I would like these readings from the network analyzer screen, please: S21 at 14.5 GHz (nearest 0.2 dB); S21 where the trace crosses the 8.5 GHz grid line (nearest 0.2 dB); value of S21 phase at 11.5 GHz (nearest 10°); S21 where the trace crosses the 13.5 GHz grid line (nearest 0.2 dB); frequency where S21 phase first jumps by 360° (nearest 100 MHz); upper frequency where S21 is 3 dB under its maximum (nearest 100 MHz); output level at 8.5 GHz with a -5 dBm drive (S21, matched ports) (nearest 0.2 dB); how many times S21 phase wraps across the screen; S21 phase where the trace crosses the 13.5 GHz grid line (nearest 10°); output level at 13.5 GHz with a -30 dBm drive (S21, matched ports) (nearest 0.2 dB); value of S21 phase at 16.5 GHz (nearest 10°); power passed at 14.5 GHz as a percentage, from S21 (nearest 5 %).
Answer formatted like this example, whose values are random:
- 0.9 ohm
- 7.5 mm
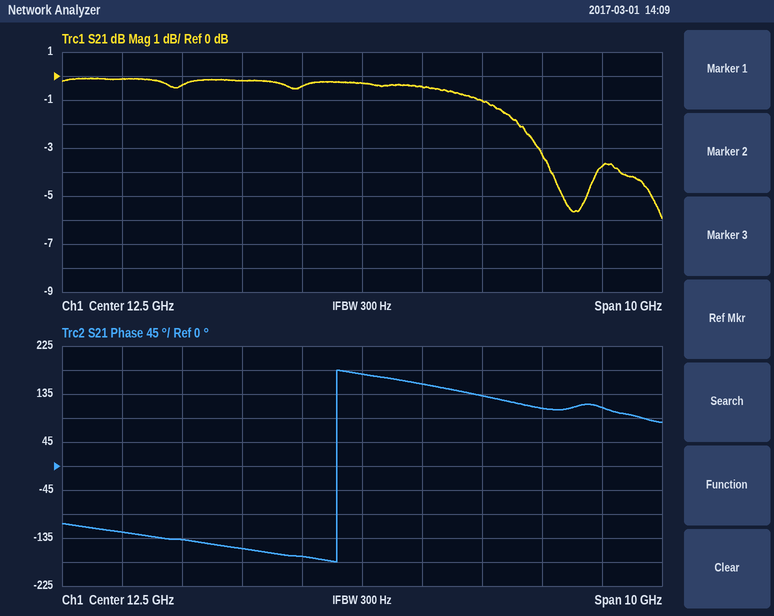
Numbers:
- -1.0 dB
- -0.2 dB
- -170°
- -0.4 dB
- 12.1 GHz
- 15.5 GHz
- -5.2 dBm
- 1
- 150°
- -30.4 dBm
- 110°
- 80 %
